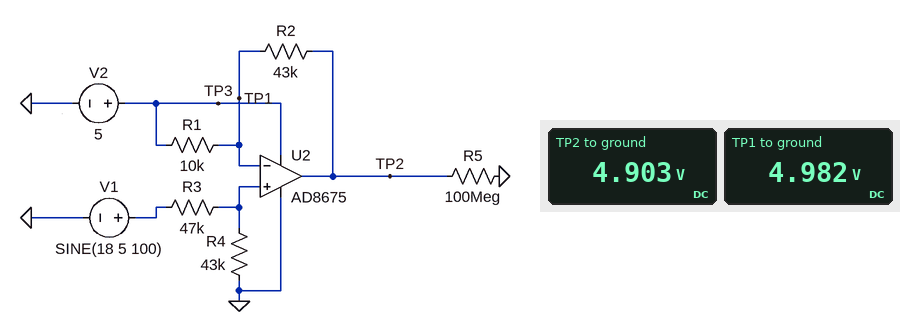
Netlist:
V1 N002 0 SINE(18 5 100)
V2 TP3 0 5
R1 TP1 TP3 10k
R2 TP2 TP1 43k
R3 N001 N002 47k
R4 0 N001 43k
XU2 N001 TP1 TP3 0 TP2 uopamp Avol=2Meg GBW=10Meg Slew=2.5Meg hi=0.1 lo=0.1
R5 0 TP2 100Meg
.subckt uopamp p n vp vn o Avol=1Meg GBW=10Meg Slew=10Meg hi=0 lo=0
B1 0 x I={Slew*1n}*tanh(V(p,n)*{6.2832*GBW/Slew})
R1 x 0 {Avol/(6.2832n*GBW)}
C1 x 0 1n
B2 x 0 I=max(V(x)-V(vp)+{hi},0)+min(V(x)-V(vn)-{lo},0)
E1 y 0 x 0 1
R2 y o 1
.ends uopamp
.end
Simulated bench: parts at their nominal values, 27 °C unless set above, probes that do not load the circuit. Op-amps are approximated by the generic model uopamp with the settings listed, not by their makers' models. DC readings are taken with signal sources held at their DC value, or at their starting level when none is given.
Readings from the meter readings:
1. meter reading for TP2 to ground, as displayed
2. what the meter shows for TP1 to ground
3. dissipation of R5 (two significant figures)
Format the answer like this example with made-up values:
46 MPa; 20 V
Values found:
4.903 V; 4.982 V; 240 nW
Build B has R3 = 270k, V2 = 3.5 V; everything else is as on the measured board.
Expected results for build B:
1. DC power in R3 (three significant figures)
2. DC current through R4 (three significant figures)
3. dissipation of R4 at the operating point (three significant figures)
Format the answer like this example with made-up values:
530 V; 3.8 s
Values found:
893 µW; 57.5 µA; 142 µW
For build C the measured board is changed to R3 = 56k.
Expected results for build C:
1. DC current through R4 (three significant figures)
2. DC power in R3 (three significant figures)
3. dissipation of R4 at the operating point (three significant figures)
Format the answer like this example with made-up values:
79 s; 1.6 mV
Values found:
182 µA; 1.85 mW; 1.42 mW
